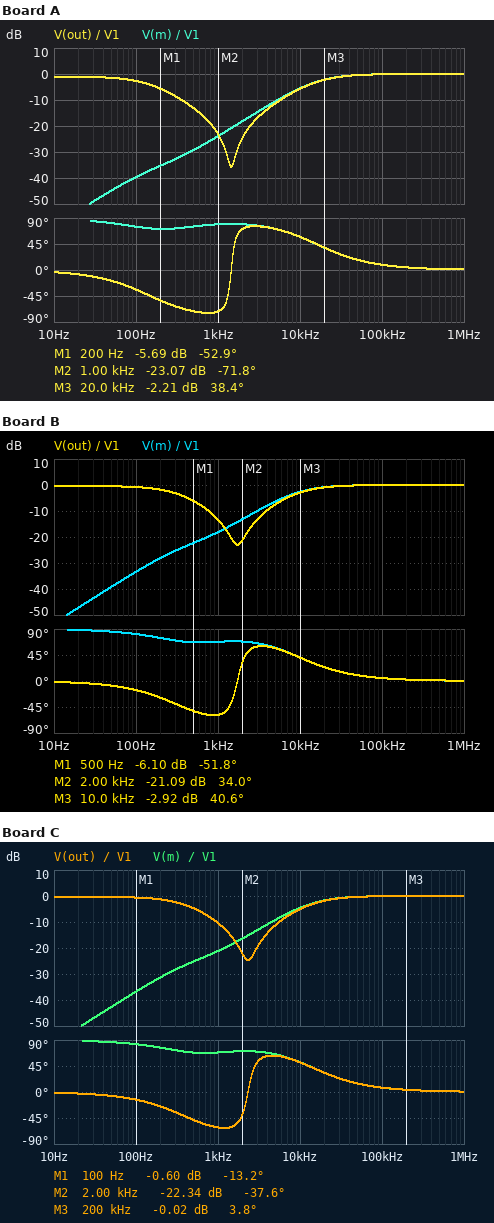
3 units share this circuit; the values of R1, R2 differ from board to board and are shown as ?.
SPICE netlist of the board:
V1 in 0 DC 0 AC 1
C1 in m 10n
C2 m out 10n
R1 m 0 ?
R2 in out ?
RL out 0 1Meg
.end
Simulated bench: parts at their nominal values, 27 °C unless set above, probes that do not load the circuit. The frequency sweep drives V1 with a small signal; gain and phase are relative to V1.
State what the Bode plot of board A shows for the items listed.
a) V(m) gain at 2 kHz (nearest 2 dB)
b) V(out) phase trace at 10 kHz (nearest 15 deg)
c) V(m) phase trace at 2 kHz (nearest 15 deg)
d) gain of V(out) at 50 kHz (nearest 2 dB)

-18 dB
60 deg
75 deg
0 dB
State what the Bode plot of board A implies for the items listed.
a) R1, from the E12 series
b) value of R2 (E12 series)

1 kΩ
120 kΩ
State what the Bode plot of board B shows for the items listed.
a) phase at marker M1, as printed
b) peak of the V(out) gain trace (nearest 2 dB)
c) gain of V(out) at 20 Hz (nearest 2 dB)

-51.8 deg
0 dB
0 dB
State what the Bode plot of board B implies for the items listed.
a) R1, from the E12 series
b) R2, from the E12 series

1.8 kΩ
47 kΩ
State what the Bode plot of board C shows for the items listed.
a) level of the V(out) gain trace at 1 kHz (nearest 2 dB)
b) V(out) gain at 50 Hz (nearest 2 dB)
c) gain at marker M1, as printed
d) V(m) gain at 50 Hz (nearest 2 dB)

-10 dB
0 dB
-0.60 dB
-42 dB
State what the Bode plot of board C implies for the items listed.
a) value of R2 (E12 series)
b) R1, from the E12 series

39 kΩ
1.2 kΩ
